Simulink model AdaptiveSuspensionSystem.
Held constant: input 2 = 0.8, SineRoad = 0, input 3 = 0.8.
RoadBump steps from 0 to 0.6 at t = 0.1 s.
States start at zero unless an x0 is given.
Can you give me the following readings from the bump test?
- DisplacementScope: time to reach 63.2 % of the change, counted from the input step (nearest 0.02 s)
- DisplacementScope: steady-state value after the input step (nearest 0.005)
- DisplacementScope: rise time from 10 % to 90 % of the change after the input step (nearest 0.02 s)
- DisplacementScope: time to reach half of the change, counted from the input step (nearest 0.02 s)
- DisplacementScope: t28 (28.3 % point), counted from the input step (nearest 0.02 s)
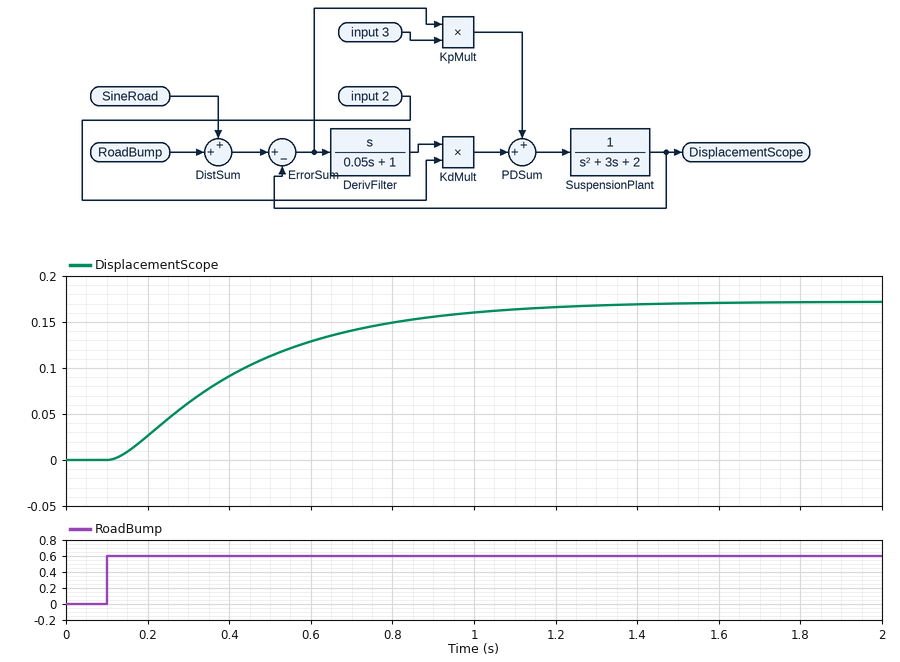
0.38 s
0.170
0.70 s
0.28 s
0.16 s
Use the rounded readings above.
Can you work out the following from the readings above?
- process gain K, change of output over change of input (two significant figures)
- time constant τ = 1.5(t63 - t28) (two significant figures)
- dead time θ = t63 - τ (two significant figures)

0.28
0.33 s
0.050 s
